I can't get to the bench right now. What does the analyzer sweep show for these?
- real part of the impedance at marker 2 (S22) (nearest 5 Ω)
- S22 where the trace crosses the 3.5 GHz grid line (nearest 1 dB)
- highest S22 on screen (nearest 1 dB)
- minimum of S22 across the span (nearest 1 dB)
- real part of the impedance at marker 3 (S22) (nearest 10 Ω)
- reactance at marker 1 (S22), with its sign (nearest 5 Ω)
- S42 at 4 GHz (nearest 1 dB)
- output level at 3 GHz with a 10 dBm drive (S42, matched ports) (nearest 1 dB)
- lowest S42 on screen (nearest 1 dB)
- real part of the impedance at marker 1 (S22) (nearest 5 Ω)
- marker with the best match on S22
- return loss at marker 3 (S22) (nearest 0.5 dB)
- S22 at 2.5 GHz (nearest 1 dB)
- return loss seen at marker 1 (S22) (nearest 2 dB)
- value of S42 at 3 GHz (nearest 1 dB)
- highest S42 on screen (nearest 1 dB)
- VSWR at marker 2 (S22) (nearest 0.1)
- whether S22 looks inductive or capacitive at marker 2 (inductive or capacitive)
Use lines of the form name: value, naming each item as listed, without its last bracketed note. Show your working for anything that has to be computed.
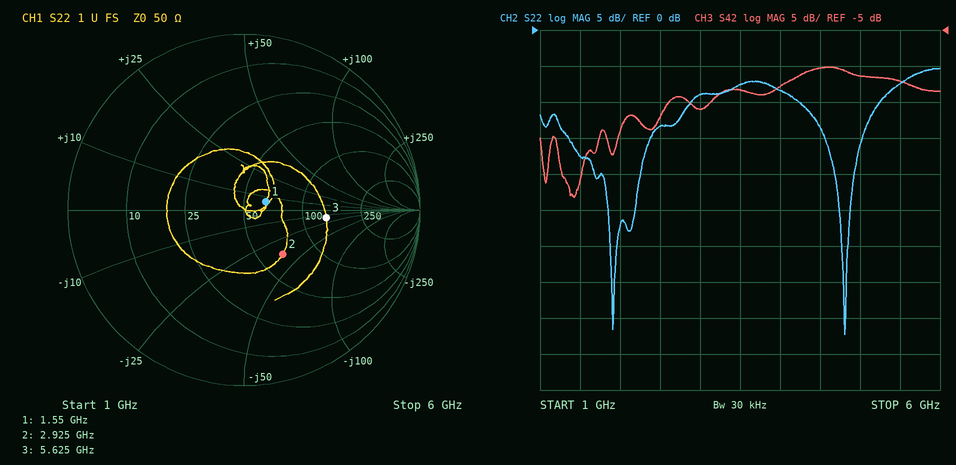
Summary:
real part of the impedance at marker 2 (S22): 65 Ω
S22 where the trace crosses the 3.5 GHz grid line: -8 dB
highest S22 on screen: -5 dB
minimum of S22 across the span: -42 dB
real part of the impedance at marker 3 (S22): 140 Ω
reactance at marker 1 (S22), with its sign: +5 Ω
S42 at 4 GHz: -13 dB
output level at 3 GHz with a 10 dBm drive (S42, matched ports): 10 dBm + (-16 dB) = -6 dBm
lowest S42 on screen: -28 dB
real part of the impedance at marker 1 (S22): 65 Ω
marker with the best match on S22: marker 1
return loss at marker 3 (S22): 6.5 dB
S22 at 2.5 GHz: -13 dB
return loss seen at marker 1 (S22): 18 dB
value of S42 at 3 GHz: -16 dB
highest S42 on screen: -10 dB
VSWR at marker 2 (S22): 2.0
whether S22 looks inductive or capacitive at marker 2: capacitive
